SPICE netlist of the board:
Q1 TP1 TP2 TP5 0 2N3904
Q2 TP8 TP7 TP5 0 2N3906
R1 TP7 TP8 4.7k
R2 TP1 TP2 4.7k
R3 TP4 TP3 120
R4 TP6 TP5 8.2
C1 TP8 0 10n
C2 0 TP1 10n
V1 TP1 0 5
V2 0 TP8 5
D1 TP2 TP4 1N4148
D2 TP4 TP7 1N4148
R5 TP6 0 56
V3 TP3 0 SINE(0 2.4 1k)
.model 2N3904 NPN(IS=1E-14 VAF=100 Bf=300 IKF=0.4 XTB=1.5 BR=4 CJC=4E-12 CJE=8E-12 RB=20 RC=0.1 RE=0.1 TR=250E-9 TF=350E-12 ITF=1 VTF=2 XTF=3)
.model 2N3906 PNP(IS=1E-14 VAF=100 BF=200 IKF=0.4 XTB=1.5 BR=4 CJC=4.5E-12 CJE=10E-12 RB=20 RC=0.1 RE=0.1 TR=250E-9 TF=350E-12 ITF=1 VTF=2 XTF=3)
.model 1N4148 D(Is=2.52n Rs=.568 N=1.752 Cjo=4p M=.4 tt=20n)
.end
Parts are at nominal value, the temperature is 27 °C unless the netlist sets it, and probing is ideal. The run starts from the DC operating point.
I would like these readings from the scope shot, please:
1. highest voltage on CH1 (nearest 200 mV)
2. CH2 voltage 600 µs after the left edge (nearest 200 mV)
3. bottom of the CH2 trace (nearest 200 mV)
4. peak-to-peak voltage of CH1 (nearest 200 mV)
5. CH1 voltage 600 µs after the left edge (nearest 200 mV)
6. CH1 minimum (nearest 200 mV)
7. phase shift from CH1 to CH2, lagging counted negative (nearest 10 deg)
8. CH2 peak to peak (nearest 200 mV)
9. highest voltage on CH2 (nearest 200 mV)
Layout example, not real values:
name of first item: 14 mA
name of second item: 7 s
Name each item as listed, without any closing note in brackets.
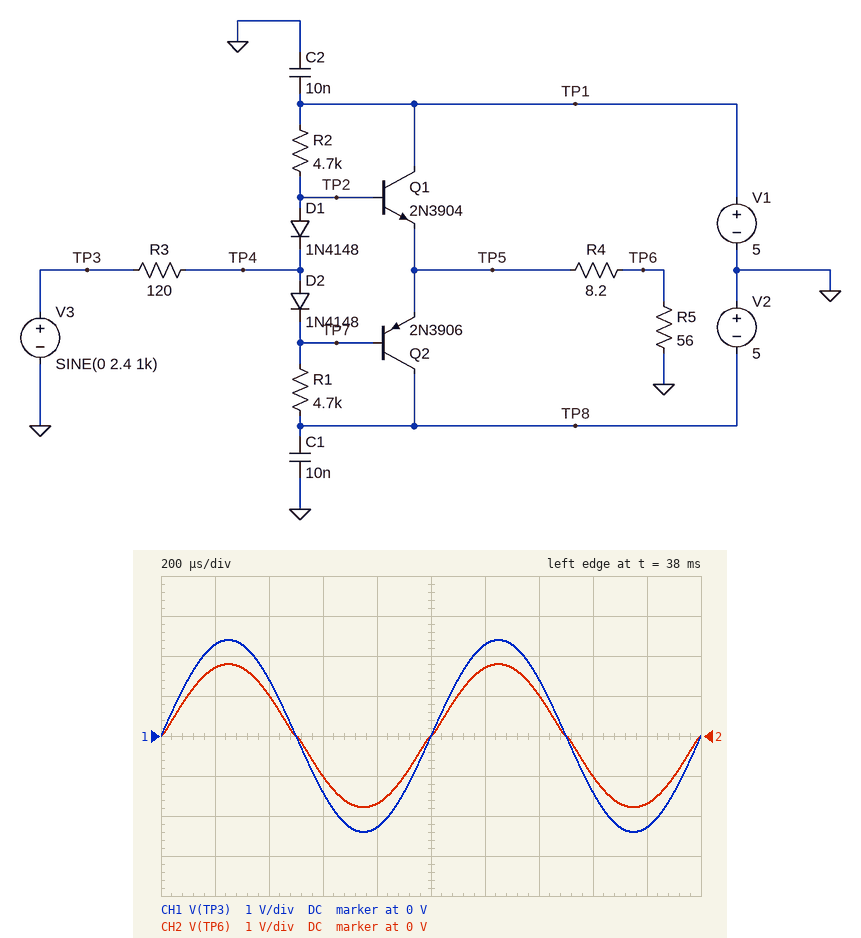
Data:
highest voltage on CH1: 2.4 V
CH2 voltage 600 µs after the left edge: -1.0 V
bottom of the CH2 trace: -1.8 V
peak-to-peak voltage of CH1: 4.8 V
CH1 voltage 600 µs after the left edge: -1.4 V
CH1 minimum: -2.4 V
phase shift from CH1 to CH2, lagging counted negative: 0 deg
CH2 peak to peak: 3.6 V
highest voltage on CH2: 1.8 V
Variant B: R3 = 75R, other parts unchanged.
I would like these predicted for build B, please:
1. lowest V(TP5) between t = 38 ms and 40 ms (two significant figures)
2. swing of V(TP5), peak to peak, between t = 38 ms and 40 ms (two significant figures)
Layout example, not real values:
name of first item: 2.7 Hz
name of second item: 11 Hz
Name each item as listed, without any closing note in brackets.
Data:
lowest V(TP5) between t = 38 ms and 40 ms: -2.1 V
swing of V(TP5), peak to peak, between t = 38 ms and 40 ms: 4.2 V
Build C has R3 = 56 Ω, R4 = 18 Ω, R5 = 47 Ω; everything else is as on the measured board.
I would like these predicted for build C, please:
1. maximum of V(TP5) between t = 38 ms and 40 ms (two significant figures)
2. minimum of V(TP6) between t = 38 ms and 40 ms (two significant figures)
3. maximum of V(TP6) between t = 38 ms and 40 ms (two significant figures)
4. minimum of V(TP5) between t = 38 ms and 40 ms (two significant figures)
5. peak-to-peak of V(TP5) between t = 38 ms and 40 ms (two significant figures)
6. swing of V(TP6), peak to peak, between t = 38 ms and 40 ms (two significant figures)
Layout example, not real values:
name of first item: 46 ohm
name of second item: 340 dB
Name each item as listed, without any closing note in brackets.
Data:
maximum of V(TP5) between t = 38 ms and 40 ms: 2.1 V
minimum of V(TP6) between t = 38 ms and 40 ms: -1.5 V
maximum of V(TP6) between t = 38 ms and 40 ms: 1.5 V
minimum of V(TP5) between t = 38 ms and 40 ms: -2.1 V
peak-to-peak of V(TP5) between t = 38 ms and 40 ms: 4.2 V
swing of V(TP6), peak to peak, between t = 38 ms and 40 ms: 3.1 V
